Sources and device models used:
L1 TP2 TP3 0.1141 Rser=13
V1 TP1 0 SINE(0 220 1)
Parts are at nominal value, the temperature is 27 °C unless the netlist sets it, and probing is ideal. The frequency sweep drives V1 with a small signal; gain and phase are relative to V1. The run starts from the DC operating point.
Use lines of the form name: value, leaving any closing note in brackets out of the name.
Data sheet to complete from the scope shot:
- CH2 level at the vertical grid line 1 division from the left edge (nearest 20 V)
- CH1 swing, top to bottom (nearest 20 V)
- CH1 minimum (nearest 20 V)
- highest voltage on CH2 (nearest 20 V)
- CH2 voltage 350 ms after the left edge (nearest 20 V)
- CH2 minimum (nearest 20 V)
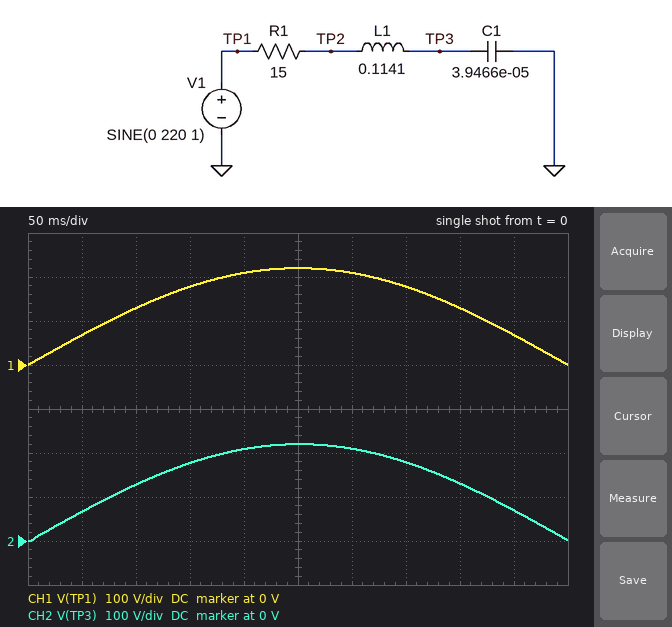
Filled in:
CH2 level at the vertical grid line 1 division from the left edge: 60 V
CH1 swing, top to bottom: 220 V
CH1 minimum: 0 V
highest voltage on CH2: 220 V
CH2 voltage 350 ms after the left edge: 180 V
CH2 minimum: 0 V
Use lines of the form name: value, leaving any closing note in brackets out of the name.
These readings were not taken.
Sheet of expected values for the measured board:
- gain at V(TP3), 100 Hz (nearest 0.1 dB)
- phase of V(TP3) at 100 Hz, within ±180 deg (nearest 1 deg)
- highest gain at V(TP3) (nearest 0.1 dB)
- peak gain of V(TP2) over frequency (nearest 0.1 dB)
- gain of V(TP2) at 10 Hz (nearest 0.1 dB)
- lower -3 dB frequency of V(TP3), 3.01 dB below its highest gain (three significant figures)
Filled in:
gain at V(TP3), 100 Hz: -0.4 dB
phase of V(TP3) at 100 Hz, within ±180 deg: -138 deg
highest gain at V(TP3): 6.0 dB
peak gain of V(TP2) over frequency: 0 dB
gain of V(TP2) at 10 Hz: 0 dB
lower -3 dB frequency of V(TP3), 3.01 dB below its highest gain: 45.1 Hz
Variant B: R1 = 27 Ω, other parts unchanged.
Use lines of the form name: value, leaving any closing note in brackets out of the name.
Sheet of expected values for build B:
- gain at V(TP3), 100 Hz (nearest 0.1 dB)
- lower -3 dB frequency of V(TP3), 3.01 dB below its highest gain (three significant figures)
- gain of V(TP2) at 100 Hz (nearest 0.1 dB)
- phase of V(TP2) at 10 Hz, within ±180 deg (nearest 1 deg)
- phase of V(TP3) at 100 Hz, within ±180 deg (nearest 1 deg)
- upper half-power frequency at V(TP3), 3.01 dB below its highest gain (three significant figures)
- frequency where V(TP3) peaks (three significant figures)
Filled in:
gain at V(TP3), 100 Hz: -2.0 dB
lower -3 dB frequency of V(TP3), 3.01 dB below its highest gain: 13.6 Hz
gain of V(TP2) at 100 Hz: -3.5 dB
phase of V(TP2) at 10 Hz, within ±180 deg: -4 deg
phase of V(TP3) at 100 Hz, within ±180 deg: -128 deg
upper half-power frequency at V(TP3), 3.01 dB below its highest gain: 89.2 Hz
frequency where V(TP3) peaks: 63.8 Hz
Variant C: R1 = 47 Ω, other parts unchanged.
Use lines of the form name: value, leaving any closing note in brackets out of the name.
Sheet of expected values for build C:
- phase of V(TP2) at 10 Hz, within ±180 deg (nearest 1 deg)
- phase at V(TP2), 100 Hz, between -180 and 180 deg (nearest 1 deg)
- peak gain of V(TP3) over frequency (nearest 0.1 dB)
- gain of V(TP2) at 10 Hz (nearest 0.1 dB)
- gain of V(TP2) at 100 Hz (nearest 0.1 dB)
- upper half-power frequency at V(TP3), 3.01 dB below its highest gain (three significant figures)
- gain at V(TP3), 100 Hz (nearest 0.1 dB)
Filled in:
phase of V(TP2) at 10 Hz, within ±180 deg: -7 deg
phase at V(TP2), 100 Hz, between -180 and 180 deg: 40 deg
peak gain of V(TP3) over frequency: 0.7 dB
gain of V(TP2) at 10 Hz: -0.1 dB
gain of V(TP2) at 100 Hz: -6.0 dB
upper half-power frequency at V(TP3), 3.01 dB below its highest gain: 85.6 Hz
gain at V(TP3), 100 Hz: -4.5 dB
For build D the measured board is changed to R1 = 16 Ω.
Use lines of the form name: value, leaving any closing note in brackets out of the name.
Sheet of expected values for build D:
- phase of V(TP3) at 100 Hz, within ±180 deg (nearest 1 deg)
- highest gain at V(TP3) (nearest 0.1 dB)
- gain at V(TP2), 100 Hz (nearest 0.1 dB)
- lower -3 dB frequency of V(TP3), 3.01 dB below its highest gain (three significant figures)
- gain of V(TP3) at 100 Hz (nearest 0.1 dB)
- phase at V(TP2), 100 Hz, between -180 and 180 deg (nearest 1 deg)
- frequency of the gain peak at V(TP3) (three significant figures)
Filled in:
phase of V(TP3) at 100 Hz, within ±180 deg: -137 deg
highest gain at V(TP3): 5.7 dB
gain at V(TP2), 100 Hz: -2.0 dB
lower -3 dB frequency of V(TP3), 3.01 dB below its highest gain: 43.4 Hz
gain of V(TP3) at 100 Hz: -0.5 dB
phase at V(TP2), 100 Hz, between -180 and 180 deg: 20 deg
frequency of the gain peak at V(TP3): 69.3 Hz
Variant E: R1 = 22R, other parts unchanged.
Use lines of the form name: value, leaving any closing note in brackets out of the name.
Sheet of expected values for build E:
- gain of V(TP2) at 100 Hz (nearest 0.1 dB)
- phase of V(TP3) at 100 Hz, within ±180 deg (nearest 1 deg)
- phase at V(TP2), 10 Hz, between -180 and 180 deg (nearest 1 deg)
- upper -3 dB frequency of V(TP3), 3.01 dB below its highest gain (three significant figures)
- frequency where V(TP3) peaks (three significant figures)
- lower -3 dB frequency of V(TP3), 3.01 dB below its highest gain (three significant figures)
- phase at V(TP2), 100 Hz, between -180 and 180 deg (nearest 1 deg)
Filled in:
gain of V(TP2) at 100 Hz: -2.8 dB
phase of V(TP3) at 100 Hz, within ±180 deg: -132 deg
phase at V(TP2), 10 Hz, between -180 and 180 deg: -3 deg
upper -3 dB frequency of V(TP3), 3.01 dB below its highest gain: 88.9 Hz
frequency where V(TP3) peaks: 66.6 Hz
lower -3 dB frequency of V(TP3), 3.01 dB below its highest gain: 31.2 Hz
phase at V(TP2), 100 Hz, between -180 and 180 deg: 26 deg
